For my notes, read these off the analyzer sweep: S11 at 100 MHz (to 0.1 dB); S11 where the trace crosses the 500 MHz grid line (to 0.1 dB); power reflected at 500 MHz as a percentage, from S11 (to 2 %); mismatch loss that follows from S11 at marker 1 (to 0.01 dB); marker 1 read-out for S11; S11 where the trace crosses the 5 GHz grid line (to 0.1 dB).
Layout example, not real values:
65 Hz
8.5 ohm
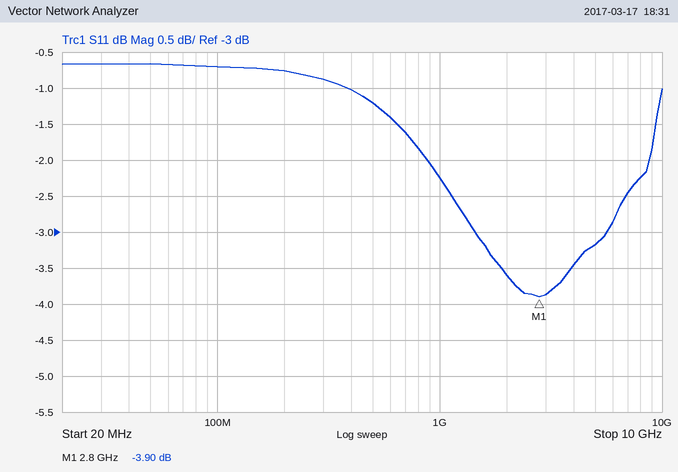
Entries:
-0.7 dB
-1.2 dB
76 %
2.27 dB
-3.90 dB
-3.2 dB
